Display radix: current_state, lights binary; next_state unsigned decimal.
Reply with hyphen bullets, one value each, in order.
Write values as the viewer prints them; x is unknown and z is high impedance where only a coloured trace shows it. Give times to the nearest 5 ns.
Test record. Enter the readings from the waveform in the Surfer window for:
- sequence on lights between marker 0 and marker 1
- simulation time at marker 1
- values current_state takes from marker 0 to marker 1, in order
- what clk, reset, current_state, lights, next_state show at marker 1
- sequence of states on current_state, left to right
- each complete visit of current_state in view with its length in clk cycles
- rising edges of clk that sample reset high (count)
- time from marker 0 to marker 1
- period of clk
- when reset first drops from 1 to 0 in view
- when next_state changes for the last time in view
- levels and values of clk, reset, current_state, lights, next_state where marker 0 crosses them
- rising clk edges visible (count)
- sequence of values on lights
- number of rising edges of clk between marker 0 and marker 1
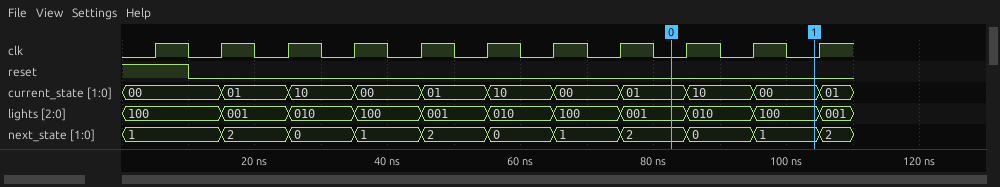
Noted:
- 001, 010, 100
- 105 ns
- 01, 10, 00
- clk=0, reset=0, current_state=00, lights=100, next_state=1
- 00, 01, 10, 00, 01, 10, 00, 01, 10, 00, 01
- 01: 1, 10: 1, 00: 1, 01: 1, 10: 1, 00: 1, 01: 1, 10: 1, 00: 1
- 1
- 20 ns
- 10 ns
- 10 ns
- 105 ns
- clk=0, reset=0, current_state=01, lights=001, next_state=2
- 11
- 100, 001, 010, 100, 001, 010, 100, 001, 010, 100, 001
- 2
